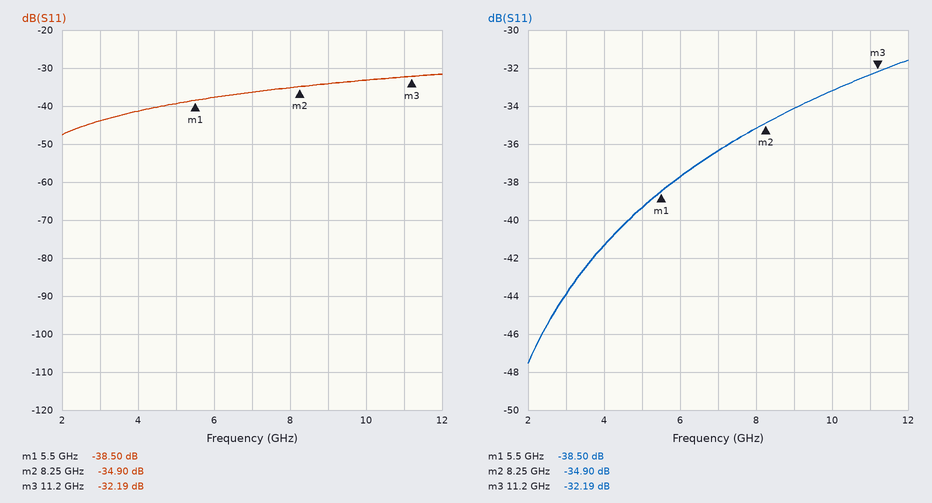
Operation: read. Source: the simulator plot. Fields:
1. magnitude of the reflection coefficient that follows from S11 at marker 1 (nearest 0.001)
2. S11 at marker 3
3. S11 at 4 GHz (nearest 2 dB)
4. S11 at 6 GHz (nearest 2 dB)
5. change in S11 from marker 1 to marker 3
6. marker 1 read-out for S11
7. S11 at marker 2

0.012
-32.19 dB
-42 dB
-38 dB
6.31 dB
-38.50 dB
-34.90 dB
